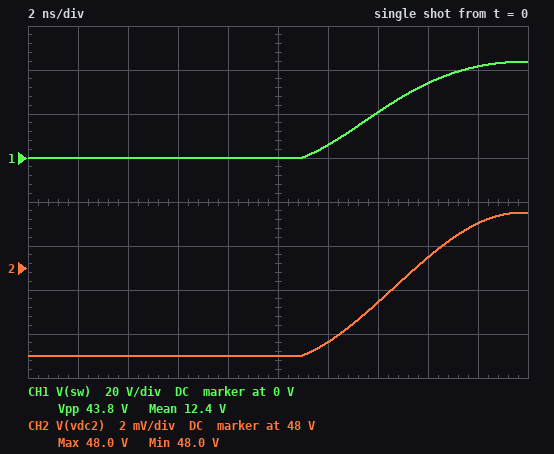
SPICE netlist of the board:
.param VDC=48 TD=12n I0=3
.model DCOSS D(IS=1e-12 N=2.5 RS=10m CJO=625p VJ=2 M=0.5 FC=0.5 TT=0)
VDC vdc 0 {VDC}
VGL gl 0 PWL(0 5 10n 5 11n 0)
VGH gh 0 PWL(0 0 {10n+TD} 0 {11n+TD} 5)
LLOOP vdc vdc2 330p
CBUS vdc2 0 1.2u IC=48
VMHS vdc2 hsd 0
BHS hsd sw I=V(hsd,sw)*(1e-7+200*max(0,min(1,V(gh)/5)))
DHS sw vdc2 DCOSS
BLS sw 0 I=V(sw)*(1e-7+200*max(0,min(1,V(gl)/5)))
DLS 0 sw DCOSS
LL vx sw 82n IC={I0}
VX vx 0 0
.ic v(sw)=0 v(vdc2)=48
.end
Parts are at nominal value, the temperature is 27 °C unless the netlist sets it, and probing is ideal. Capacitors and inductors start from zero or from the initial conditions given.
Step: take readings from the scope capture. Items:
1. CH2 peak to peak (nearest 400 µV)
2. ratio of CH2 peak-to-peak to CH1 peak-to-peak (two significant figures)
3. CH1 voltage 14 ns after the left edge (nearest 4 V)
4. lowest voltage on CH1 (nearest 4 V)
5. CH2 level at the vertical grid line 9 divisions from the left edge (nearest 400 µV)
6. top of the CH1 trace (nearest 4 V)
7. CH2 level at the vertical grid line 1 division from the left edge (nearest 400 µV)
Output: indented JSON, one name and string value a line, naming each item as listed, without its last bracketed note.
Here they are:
{
  "CH2 peak to peak": "6.4 mV",
  "ratio of CH2 peak-to-peak to CH1 peak-to-peak": "0.00015",
  "CH1 voltage 14 ns after the left edge": "20 V",
  "lowest voltage on CH1": "0 V",
  "CH2 level at the vertical grid line 9 divisions from the left edge": "48.0060 V",
  "top of the CH1 trace": "44 V",
  "CH2 level at the vertical grid line 1 division from the left edge": "48.0000 V"
}
